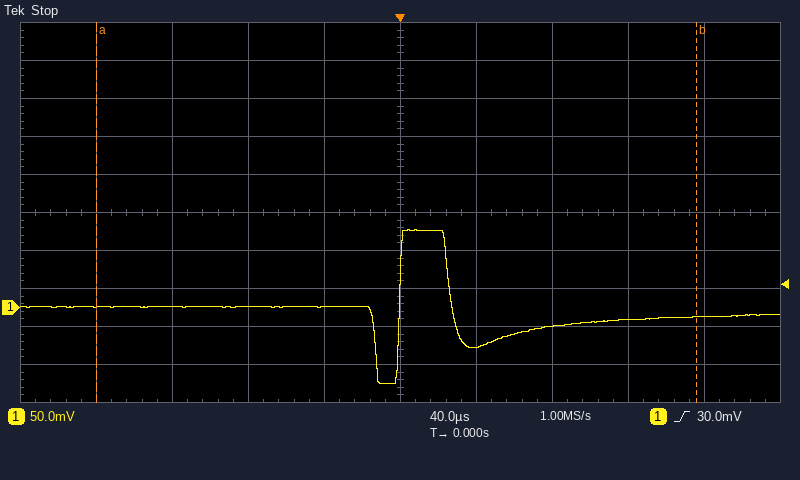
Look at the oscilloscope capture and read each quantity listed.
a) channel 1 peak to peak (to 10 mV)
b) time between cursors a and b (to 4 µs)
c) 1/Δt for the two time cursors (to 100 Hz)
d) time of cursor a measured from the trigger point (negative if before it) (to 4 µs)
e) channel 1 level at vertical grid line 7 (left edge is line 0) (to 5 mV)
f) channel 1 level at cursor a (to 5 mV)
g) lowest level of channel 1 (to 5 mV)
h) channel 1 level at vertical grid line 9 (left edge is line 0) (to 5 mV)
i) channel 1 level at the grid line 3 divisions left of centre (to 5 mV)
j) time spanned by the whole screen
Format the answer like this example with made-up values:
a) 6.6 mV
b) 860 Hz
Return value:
a) 200 mV
b) 316 µs
c) 3.2 kHz
d) -160 µs
e) -25 mV
f) 0 mV
g) -100 mV
h) -10 mV
i) 0 mV
j) 400 µs
